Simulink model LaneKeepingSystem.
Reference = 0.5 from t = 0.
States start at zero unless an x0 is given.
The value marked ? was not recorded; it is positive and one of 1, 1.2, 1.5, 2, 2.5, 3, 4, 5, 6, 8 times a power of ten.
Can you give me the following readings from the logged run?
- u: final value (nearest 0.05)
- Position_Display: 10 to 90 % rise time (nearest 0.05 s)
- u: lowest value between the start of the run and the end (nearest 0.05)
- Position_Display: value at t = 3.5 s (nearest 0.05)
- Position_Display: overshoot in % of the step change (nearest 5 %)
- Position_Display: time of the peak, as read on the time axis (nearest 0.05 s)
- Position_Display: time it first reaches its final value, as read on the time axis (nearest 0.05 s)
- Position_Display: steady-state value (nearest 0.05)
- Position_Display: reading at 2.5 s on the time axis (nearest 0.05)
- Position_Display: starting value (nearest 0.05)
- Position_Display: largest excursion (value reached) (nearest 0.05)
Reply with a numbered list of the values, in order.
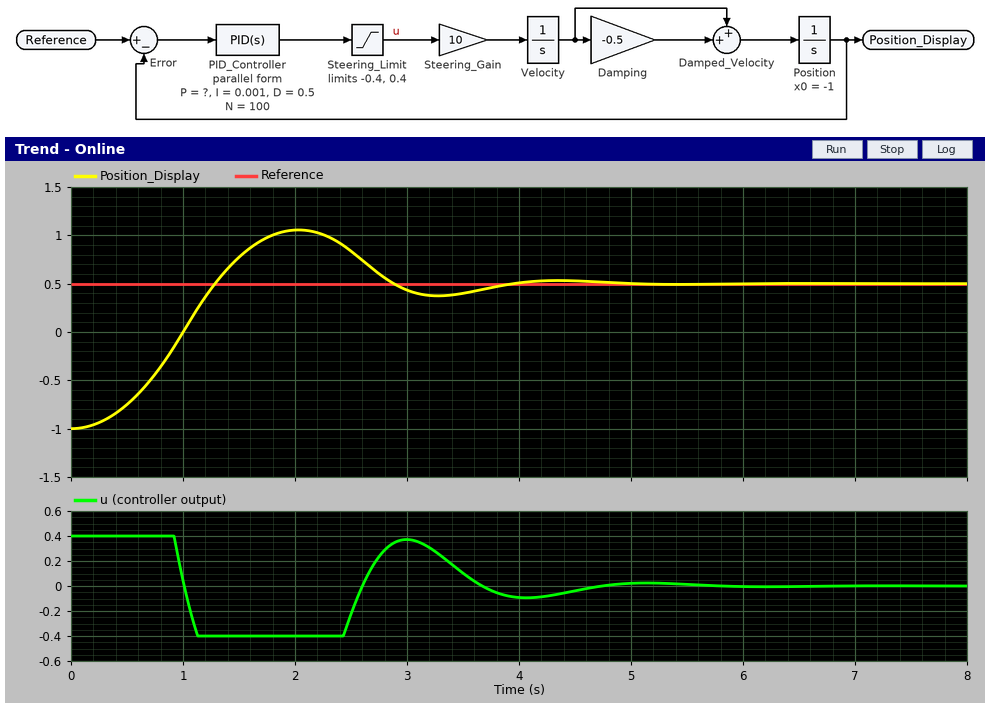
1. 0.00
2. 0.80 s
3. -0.40
4. 0.40
5. 35 %
6. 2.05 s
7. 1.30 s
8. 0.50
9. 0.85
10. -1.00
11. 1.05
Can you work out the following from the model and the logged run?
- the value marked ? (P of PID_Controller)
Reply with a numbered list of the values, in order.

1. 2
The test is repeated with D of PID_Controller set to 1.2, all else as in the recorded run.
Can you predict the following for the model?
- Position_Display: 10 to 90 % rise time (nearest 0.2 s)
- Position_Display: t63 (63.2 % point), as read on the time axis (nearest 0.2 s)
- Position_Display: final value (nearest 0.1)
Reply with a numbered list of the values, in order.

1. 1.2 s
2. 1.0 s
3. 0.5
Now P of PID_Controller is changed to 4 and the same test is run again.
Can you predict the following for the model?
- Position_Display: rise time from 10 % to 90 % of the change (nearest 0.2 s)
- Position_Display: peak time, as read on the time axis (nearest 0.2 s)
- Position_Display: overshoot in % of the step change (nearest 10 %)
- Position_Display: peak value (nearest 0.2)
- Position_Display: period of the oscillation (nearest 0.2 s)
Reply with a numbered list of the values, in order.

1. 0.8 s
2. 2.2 s
3. 60 %
4. 1.4
5. 3.0 s
